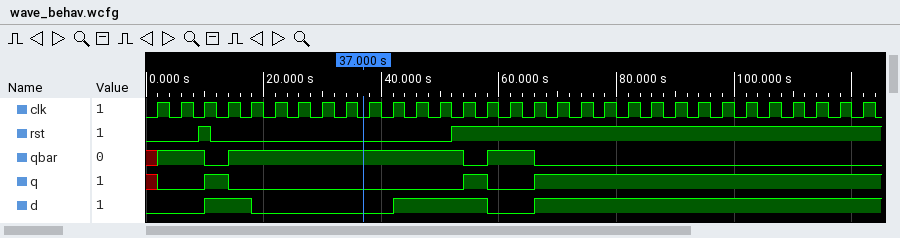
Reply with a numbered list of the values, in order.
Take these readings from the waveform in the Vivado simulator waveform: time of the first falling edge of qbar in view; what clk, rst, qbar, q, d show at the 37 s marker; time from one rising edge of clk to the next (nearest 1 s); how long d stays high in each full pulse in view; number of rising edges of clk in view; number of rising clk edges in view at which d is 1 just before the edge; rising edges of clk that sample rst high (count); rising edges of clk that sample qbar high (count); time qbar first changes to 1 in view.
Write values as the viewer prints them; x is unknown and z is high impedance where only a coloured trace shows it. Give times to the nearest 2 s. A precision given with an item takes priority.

1. 10 s
2. clk=0, rst=0, qbar=1, q=0, d=0
3. 4 s
4. 8 s, 16 s
5. 31
6. 20
7. 19
8. 14
9. 2 s
